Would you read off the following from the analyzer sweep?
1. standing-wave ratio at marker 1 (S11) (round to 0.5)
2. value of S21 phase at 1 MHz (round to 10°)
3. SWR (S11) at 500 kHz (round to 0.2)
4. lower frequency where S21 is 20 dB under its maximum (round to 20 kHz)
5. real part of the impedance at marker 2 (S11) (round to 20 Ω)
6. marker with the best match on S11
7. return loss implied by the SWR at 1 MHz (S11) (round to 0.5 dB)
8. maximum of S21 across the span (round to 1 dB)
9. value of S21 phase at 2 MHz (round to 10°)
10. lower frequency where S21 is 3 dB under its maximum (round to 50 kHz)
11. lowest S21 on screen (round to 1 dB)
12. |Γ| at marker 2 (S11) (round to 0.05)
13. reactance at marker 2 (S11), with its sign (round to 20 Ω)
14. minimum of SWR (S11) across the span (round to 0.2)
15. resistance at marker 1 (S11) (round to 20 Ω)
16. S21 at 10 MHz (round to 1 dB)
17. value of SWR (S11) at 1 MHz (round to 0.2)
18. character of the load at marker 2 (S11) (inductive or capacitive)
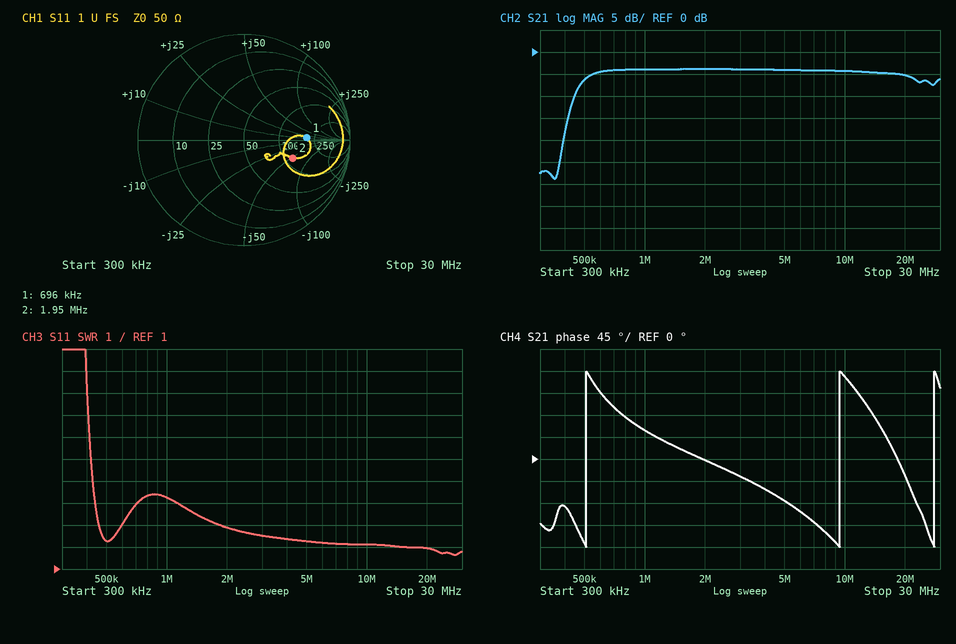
4.0
60°
2.2
380 kHz
120 Ω
marker 2
4.0 dB
-4 dB
0°
500 kHz
-29 dB
0.50
-60 Ω
1.6
200 Ω
-4 dB
4.2
capacitive
